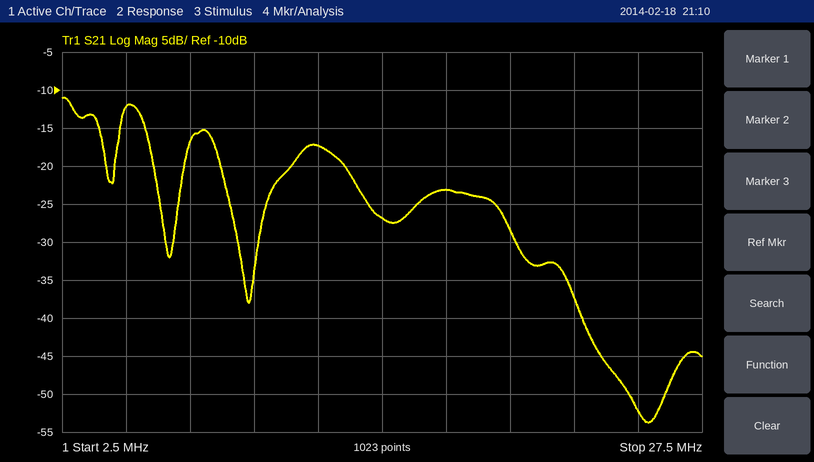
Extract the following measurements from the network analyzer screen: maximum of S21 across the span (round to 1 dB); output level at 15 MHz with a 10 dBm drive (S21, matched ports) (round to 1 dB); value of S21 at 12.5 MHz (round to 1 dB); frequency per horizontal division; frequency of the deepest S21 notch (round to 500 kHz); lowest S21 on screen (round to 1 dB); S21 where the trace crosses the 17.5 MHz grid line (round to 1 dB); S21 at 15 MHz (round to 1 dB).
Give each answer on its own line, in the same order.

-11 dB
-17 dBm
-17 dB
2.5 MHz
25.5 MHz
-54 dB
-23 dB
-27 dB
